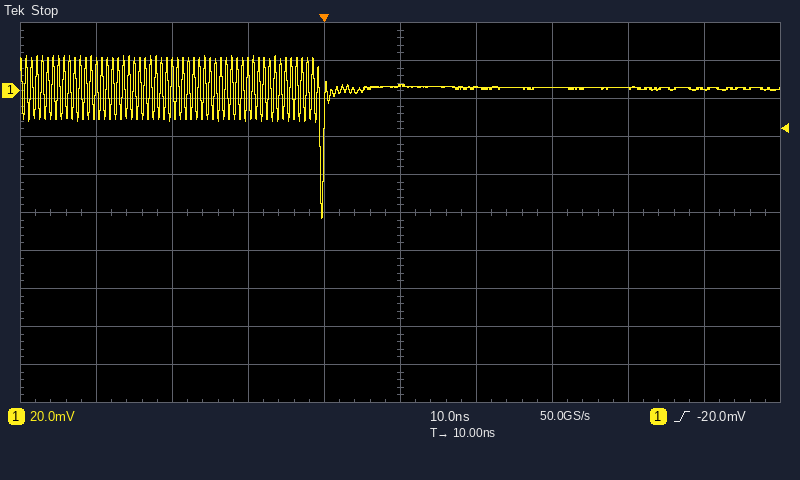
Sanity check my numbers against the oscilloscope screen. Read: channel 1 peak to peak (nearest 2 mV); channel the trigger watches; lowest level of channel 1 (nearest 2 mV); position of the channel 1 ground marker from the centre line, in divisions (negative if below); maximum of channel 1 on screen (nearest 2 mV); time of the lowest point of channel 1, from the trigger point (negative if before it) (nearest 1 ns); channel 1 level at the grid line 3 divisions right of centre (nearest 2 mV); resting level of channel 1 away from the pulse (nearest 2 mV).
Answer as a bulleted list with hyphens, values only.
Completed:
- 86 mV
- channel 1
- -68 mV
- +3.2 div
- 18 mV
- 0 ns
- 2 mV
- 2 mV
